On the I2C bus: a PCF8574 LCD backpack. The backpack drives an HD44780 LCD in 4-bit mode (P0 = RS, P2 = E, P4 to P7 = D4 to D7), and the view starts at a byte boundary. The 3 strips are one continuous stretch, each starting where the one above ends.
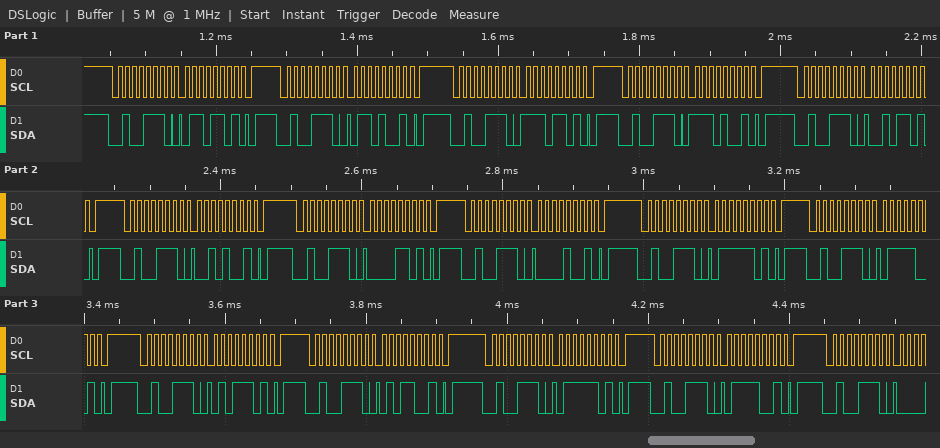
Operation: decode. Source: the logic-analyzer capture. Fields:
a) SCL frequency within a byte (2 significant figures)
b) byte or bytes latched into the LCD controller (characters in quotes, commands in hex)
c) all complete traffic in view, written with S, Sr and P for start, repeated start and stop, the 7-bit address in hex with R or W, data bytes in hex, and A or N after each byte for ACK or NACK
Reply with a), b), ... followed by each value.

a) 100 kHz
b) 'n' ' ' 'u'
c) S 27W A 6D A P S 27W A 69 A P S 27W A ED A P S 27W A E9 A P S 27W A 2D A P S 27W A 29 A P S 27W A 0D A P S 27W A 09 A P S 27W A 7D A P S 27W A 79 A P S 27W A 5D A P S 27W A 59 A P S 27W A 7D A P S 27W A 79 A P S 27W A
